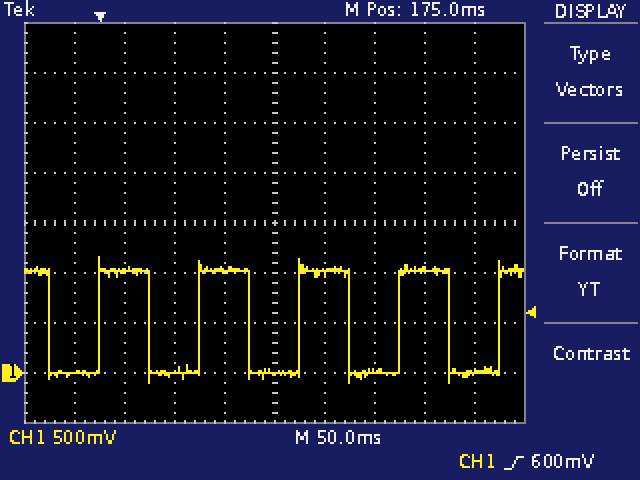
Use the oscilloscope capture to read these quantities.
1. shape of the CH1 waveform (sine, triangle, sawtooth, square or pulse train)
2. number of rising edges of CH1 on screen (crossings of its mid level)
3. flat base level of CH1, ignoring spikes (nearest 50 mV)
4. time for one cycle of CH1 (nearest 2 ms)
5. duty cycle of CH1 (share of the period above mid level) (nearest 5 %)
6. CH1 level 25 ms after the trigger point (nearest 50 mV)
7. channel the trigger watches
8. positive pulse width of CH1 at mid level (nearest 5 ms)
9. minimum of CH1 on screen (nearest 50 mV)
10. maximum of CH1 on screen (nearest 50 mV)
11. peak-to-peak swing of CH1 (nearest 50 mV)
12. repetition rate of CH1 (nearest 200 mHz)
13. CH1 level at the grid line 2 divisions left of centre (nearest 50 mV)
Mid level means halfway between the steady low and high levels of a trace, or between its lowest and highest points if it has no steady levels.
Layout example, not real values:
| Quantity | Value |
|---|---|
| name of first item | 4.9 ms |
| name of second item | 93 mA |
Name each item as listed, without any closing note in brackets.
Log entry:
| Quantity | Value |
|---|---|
| shape of the CH1 waveform | square |
| number of rising edges of CH1 on screen | 5 |
| flat base level of CH1, ignoring spikes | 0 mV |
| time for one cycle of CH1 | 100 ms |
| duty cycle of CH1 (share of the period above mid level) | 50 % |
| CH1 level 25 ms after the trigger point | 1.00 V |
| channel the trigger watches | CH1 |
| positive pulse width of CH1 at mid level | 50 ms |
| minimum of CH1 on screen | -100 mV |
| maximum of CH1 on screen | 1.15 V |
| peak-to-peak swing of CH1 | 1.25 V |
| repetition rate of CH1 | 10.0 Hz |
| CH1 level at the grid line 2 divisions left of centre | 0 mV |
